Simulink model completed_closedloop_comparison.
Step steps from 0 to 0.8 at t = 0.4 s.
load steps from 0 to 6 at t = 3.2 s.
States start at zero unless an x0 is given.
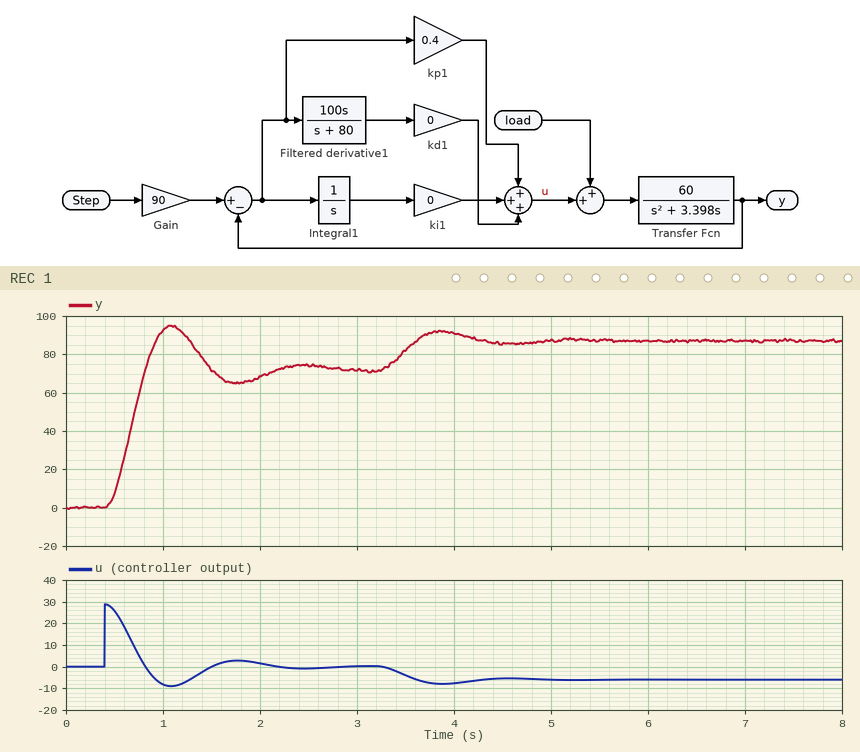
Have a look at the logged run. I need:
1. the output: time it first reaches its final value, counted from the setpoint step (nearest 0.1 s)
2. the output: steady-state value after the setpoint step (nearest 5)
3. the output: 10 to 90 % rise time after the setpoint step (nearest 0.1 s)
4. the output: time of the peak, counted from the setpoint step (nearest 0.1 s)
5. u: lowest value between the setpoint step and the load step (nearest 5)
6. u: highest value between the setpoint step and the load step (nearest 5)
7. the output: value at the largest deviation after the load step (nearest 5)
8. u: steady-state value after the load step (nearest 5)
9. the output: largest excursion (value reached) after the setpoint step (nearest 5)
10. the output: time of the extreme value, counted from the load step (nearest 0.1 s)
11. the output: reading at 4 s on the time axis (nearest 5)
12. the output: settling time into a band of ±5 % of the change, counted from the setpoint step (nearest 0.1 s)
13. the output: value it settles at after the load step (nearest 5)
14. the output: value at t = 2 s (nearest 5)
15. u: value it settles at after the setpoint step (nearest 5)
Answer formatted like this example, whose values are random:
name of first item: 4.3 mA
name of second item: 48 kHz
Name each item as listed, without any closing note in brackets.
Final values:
the output: time it first reaches its final value, counted from the setpoint step: 0.4 s
the output: steady-state value after the setpoint step: 70
the output: 10 to 90 % rise time after the setpoint step: 0.3 s
the output: time of the peak, counted from the setpoint step: 0.7 s
u: lowest value between the setpoint step and the load step: -10
u: highest value between the setpoint step and the load step: 30
the output: value at the largest deviation after the load step: 90
u: steady-state value after the load step: -5
the output: largest excursion (value reached) after the setpoint step: 95
the output: time of the extreme value, counted from the load step: 0.7 s
the output: reading at 4 s on the time axis: 90
the output: settling time into a band of ±5 % of the change, counted from the setpoint step: 1.6 s
the output: value it settles at after the load step: 85
the output: value at t = 2 s: 70
u: value it settles at after the setpoint step: 0
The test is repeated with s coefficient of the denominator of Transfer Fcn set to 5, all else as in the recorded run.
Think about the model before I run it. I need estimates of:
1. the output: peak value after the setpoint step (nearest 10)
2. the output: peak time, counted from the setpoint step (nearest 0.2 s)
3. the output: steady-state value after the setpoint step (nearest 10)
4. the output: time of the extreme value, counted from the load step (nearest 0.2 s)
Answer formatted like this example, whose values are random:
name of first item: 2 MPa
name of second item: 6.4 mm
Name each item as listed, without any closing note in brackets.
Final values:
the output: peak value after the setpoint step: 80
the output: peak time, counted from the setpoint step: 0.8 s
the output: steady-state value after the setpoint step: 70
the output: time of the extreme value, counted from the load step: 0.8 s
